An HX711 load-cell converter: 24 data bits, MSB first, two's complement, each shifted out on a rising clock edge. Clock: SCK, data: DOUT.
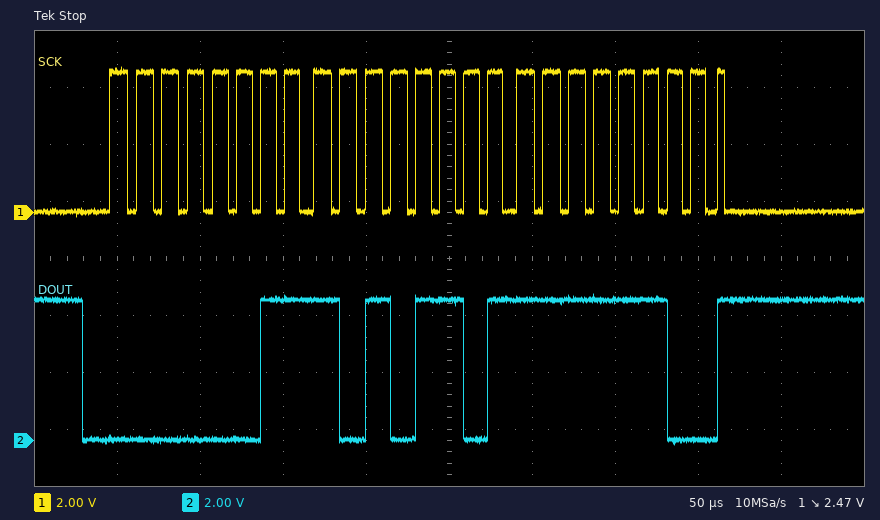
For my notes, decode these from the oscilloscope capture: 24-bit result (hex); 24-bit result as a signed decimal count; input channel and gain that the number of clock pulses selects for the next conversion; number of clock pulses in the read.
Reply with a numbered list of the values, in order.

1. 0x03ADFC
2. 241148
3. channel A, gain 128
4. 25
